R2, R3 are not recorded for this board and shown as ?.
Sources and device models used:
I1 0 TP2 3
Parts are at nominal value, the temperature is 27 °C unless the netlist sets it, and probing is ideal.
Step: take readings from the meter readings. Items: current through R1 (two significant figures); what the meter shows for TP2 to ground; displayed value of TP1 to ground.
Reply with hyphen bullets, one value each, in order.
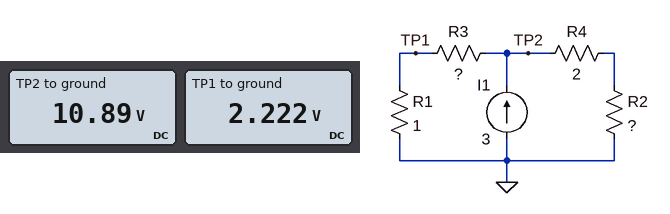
- 2.2 A
- 10.89 V
- 2.222 V
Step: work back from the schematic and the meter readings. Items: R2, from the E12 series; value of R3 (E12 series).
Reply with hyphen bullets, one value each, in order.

- 12 Ω
- 3.9 Ω
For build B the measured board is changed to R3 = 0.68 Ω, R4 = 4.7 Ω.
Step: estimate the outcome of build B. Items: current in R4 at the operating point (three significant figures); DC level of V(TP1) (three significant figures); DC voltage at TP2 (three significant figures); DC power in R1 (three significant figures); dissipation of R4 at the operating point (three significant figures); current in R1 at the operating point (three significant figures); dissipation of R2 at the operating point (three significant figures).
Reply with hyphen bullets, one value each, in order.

- 274 mA
- 2.73 V
- 4.58 V
- 7.43 W
- 353 mW
- 2.73 A
- 902 mW
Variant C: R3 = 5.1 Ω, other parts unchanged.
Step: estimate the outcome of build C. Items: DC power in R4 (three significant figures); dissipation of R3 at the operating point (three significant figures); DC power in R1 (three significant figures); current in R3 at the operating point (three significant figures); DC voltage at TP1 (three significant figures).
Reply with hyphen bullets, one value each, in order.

- 1.66 W
- 22.3 W
- 4.37 W
- 2.09 A
- 2.09 V
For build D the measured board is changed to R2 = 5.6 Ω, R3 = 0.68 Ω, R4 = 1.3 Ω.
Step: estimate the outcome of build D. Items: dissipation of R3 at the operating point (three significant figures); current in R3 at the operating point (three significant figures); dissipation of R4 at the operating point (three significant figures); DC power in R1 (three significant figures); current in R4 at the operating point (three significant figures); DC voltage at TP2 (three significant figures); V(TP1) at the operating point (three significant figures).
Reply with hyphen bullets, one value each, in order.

- 3.96 W
- 2.41 A
- 449 mW
- 5.82 W
- 587 mA
- 4.05 V
- 2.41 V
